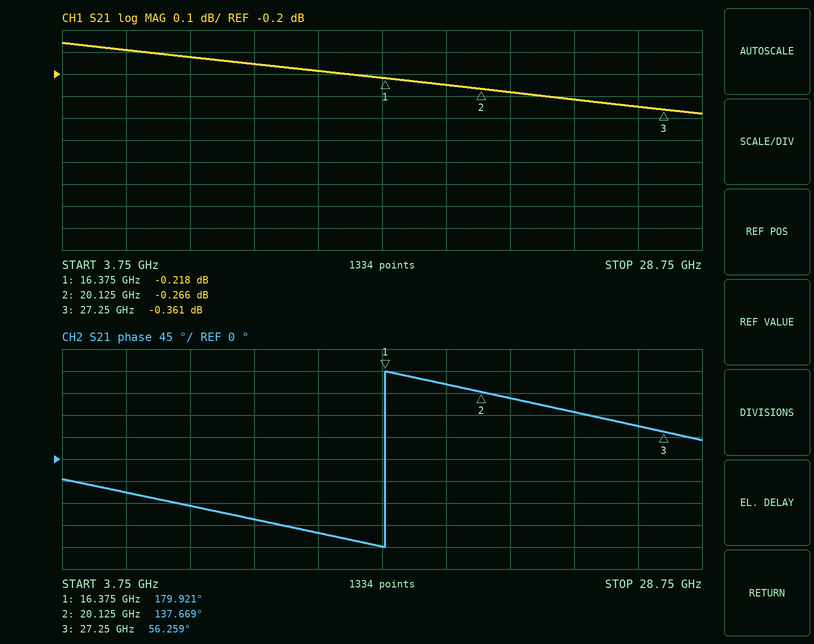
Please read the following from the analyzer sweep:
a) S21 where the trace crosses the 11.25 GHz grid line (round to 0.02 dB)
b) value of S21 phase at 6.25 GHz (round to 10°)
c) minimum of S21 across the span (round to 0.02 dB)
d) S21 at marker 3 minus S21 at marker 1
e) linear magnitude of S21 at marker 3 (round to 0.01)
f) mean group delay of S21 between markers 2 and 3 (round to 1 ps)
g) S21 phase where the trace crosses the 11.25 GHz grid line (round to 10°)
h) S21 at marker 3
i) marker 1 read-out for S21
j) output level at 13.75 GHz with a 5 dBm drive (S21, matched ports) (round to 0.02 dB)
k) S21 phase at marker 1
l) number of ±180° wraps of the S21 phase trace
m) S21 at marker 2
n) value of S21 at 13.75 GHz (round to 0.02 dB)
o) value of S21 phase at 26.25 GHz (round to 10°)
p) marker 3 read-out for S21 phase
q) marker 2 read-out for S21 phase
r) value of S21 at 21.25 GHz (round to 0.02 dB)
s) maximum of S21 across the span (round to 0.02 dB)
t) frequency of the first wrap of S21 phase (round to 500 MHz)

-0.16 dB
-70°
-0.38 dB
-0.143 dB
0.96
32 ps
-120°
-0.361 dB
-0.218 dB
4.82 dBm
179.921°
1
-0.266 dB
-0.18 dB
70°
56.259°
137.669°
-0.28 dB
-0.06 dB
16.5 GHz
